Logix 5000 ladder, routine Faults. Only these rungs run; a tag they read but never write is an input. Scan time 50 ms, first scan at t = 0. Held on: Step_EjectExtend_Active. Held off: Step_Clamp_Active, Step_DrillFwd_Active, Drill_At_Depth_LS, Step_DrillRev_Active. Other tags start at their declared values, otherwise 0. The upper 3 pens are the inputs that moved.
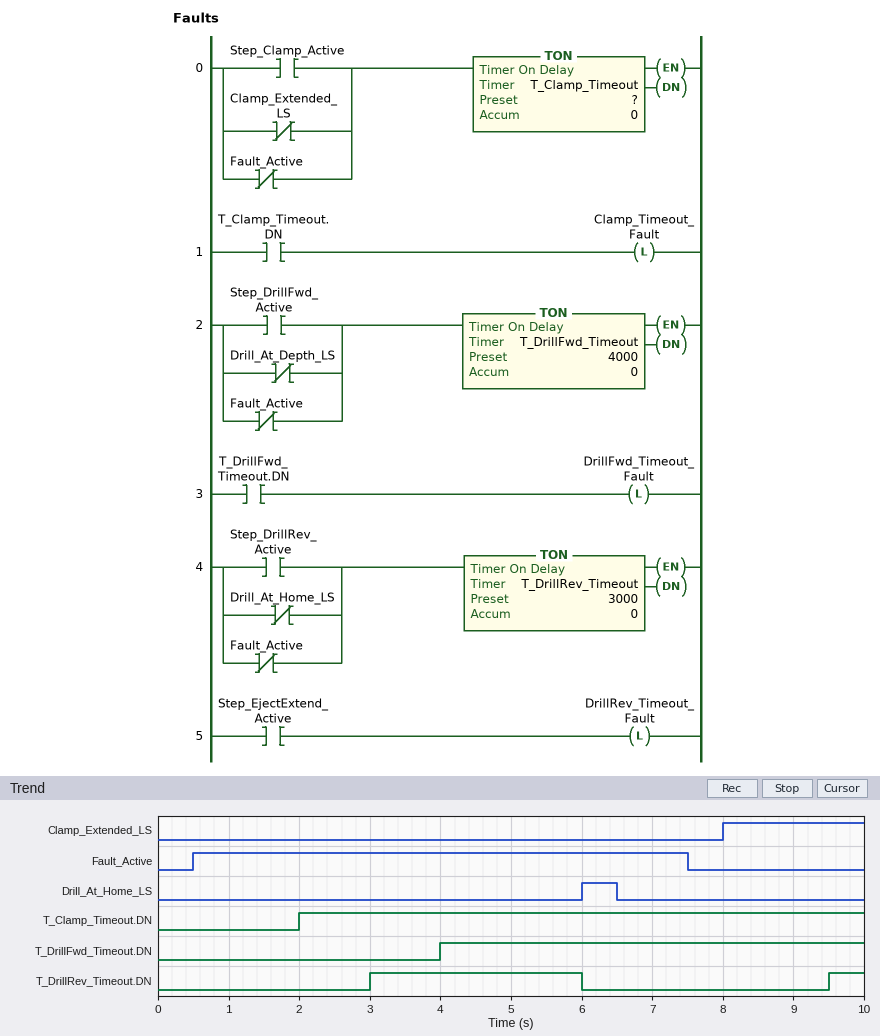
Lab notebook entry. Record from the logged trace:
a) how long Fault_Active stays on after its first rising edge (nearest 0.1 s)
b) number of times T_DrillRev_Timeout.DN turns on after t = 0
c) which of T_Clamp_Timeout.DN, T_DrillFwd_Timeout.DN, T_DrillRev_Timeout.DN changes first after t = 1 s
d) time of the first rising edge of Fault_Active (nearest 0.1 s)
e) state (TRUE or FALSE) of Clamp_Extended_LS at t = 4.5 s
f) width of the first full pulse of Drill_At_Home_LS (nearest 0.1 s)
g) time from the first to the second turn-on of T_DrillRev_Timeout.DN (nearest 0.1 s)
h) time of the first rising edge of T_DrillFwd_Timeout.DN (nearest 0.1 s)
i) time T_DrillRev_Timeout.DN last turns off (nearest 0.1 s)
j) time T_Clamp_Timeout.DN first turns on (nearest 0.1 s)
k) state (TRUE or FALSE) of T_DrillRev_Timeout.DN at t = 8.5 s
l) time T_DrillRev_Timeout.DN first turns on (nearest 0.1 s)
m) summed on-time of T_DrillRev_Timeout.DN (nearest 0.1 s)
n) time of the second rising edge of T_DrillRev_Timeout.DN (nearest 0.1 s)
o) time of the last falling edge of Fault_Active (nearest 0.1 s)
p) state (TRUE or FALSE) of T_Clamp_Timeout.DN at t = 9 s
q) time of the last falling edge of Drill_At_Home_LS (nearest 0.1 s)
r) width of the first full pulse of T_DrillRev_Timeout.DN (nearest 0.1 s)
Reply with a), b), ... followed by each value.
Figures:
a) 7.0 s
b) 2
c) T_Clamp_Timeout.DN
d) 0.5 s
e) FALSE
f) 0.5 s
g) 6.5 s
h) 4.0 s
i) 6.0 s
j) 2.0 s
k) FALSE
l) 3.0 s
m) 3.5 s
n) 9.5 s
o) 7.5 s
p) TRUE
q) 6.5 s
r) 3.0 s
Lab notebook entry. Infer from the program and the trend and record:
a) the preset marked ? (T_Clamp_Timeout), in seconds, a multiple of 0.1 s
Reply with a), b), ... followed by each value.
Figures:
a) 2.0 s
